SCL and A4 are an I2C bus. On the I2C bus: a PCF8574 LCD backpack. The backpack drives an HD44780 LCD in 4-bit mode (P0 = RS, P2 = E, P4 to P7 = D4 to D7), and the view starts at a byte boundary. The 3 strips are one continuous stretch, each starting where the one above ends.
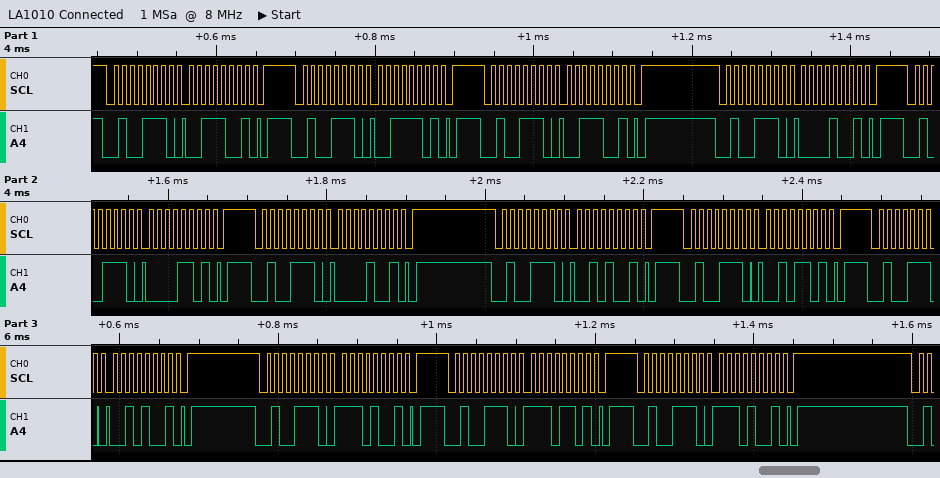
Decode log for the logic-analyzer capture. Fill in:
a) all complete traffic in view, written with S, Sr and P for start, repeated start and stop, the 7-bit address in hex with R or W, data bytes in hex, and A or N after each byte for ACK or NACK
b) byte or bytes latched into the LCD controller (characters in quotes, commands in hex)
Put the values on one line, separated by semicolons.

S 27W A 39 A P S 27W A 3D A P S 27W A 39 A P S 27W A 09 A P S 27W A 0D A P S 27W A 09 A P S 27W A 29 A P S 27W A 2D A P S 27W A 29 A P S 27W A E9 A P S 27W A ED A P S 27W A E9 A P; '0' '.'
